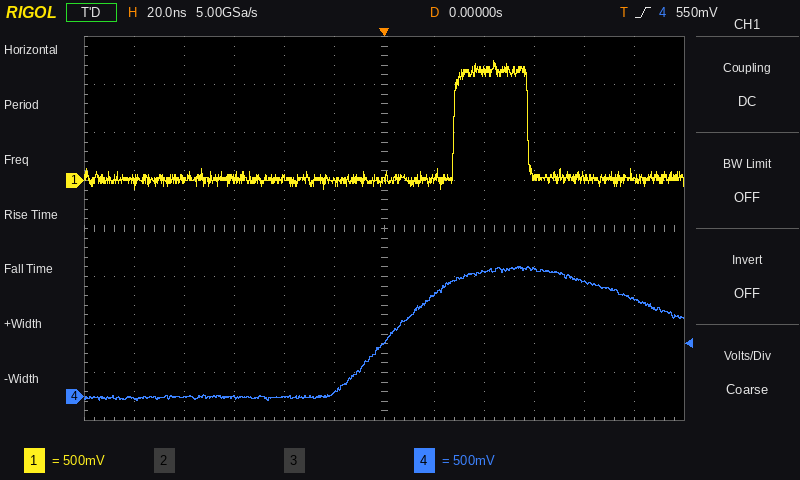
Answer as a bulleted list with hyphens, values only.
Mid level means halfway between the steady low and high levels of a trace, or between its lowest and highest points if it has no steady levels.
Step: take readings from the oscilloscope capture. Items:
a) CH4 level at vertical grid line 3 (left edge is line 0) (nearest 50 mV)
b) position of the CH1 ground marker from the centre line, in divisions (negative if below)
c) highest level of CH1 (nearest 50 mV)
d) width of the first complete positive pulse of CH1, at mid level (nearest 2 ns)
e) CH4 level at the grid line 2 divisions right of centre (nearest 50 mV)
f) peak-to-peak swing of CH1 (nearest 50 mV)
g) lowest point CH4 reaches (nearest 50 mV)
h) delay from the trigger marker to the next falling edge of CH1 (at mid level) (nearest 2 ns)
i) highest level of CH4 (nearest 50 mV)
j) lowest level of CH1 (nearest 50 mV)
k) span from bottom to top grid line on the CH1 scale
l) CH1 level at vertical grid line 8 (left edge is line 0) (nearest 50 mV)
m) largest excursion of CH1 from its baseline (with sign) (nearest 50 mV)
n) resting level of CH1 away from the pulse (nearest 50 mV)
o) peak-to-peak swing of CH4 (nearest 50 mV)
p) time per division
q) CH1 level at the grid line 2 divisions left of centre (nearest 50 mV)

- 0 mV
- +1.0 div
- 1.25 V
- 30 ns
- 1.30 V
- 1.35 V
- -50 mV
- 58 ns
- 1.35 V
- -100 mV
- 4 V
- 1.15 V
- +1.25 V
- 0 mV
- 1.40 V
- 20 ns
- 0 mV
